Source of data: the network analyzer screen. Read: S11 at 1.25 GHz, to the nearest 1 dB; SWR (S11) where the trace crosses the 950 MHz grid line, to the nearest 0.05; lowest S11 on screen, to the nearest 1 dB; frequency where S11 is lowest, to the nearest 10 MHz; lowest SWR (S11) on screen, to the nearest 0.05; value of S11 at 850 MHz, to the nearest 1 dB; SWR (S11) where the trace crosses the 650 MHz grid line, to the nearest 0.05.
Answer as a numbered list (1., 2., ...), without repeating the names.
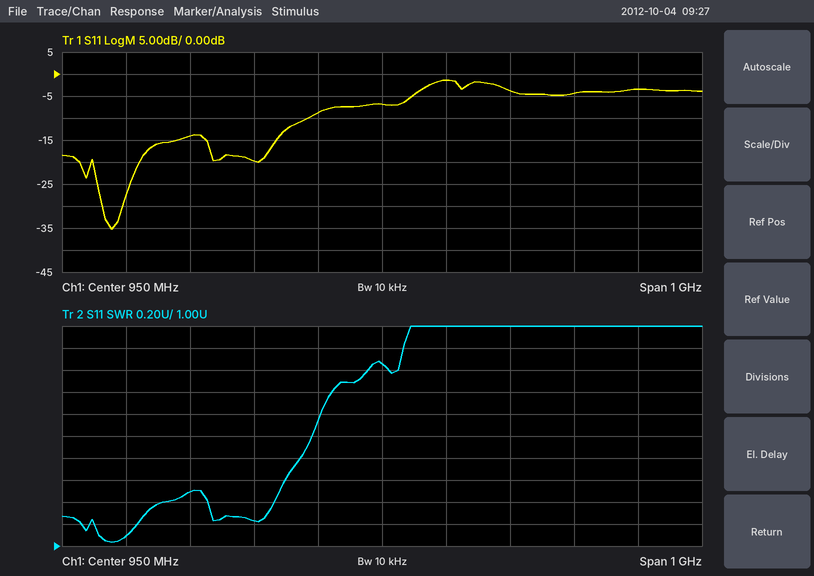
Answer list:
1. -4 dB
2. 2.65
3. -35 dB
4. 530 MHz
5. 1.05
6. -9 dB
7. 1.50
